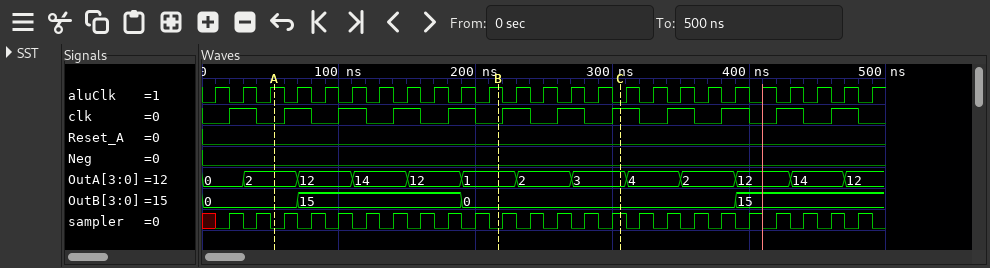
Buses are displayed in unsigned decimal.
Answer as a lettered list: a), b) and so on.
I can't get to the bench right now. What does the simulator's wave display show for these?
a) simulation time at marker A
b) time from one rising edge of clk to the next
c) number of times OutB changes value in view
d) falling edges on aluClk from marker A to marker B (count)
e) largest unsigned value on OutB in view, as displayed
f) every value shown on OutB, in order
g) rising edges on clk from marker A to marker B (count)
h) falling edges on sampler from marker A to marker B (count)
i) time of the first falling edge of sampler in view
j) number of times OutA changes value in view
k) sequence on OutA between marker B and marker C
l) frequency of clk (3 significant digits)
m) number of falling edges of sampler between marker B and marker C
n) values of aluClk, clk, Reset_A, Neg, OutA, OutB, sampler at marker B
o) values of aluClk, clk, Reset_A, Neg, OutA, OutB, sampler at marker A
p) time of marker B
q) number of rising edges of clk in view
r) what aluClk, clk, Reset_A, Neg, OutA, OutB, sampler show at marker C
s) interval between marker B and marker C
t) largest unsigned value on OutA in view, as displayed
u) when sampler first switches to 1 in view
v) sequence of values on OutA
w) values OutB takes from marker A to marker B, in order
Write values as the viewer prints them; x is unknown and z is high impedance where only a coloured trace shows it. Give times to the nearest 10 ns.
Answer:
a) 50 ns
b) 40 ns
c) 3
d) 8
e) 15
f) 0, 15, 0, 15
g) 4
h) 8
i) 30 ns
j) 12
k) 1, 2, 3
l) 25.0 MHz
m) 4
n) aluClk=1, clk=0, Reset_A=0, Neg=0, OutA=1, OutB=0, sampler=0
o) aluClk=1, clk=0, Reset_A=0, Neg=0, OutA=2, OutB=0, sampler=0
p) 220 ns
q) 12
r) aluClk=0, clk=1, Reset_A=0, Neg=0, OutA=3, OutB=0, sampler=1
s) 90 ns
t) 14
u) 20 ns
v) 0, 2, 12, 14, 12, 1, 2, 3, 4, 2, 12, 14, 12
w) 0, 15, 0
